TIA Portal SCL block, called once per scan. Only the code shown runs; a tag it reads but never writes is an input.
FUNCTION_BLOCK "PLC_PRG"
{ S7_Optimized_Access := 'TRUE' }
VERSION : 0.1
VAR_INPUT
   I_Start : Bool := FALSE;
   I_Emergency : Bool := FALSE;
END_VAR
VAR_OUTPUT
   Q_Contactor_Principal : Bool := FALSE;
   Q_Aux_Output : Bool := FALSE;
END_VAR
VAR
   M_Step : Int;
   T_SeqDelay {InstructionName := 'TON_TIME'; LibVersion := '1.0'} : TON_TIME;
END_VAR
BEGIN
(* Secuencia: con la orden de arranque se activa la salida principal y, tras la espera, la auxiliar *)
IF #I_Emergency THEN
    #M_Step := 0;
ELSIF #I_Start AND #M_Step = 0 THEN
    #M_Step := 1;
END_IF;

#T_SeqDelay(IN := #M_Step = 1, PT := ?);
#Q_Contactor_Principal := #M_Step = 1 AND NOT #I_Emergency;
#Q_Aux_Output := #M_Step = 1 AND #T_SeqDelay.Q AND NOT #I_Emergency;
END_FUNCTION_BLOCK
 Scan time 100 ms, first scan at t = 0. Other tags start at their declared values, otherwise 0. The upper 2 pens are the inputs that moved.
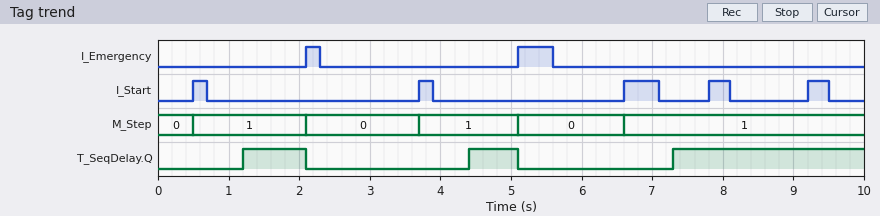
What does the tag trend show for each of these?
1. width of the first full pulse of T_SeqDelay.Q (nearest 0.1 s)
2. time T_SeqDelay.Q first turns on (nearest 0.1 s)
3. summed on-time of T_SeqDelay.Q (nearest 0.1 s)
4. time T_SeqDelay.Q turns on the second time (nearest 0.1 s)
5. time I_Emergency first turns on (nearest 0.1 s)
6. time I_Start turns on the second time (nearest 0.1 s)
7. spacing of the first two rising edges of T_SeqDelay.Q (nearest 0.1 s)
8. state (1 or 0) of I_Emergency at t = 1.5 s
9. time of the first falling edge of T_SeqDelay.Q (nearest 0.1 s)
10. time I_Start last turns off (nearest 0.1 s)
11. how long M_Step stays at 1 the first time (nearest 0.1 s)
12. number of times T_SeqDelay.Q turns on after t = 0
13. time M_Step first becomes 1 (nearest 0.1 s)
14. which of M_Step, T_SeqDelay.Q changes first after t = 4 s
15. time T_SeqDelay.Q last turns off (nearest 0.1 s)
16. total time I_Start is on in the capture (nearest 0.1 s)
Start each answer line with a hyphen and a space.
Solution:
- 0.9 s
- 1.2 s
- 4.3 s
- 4.4 s
- 2.1 s
- 3.7 s
- 3.2 s
- 0
- 2.1 s
- 9.5 s
- 1.6 s
- 3
- 0.5 s
- T_SeqDelay.Q
- 5.1 s
- 1.5 s
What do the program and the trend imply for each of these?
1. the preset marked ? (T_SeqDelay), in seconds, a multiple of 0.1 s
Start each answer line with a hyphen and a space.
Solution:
- 0.7 s
